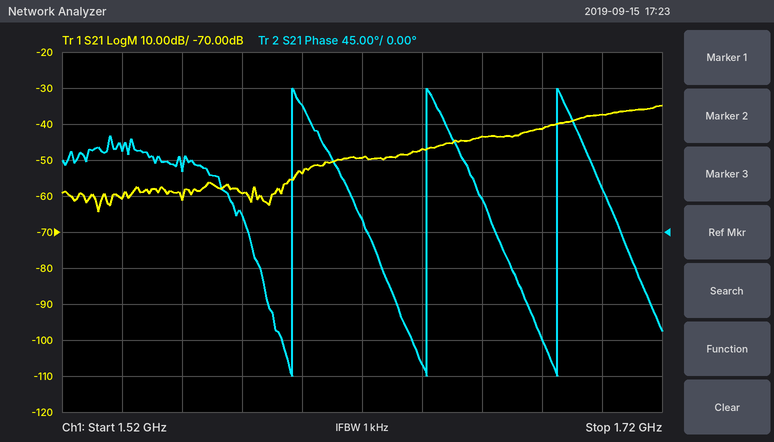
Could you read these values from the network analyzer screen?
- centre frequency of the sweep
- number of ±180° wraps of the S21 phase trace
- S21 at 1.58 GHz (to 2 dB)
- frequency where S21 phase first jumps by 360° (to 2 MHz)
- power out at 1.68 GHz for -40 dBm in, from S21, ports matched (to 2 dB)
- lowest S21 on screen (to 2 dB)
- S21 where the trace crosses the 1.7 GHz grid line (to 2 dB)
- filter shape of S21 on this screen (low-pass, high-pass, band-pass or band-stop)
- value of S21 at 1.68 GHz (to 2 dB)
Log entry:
1.62 GHz
3
-60 dB
1.596 GHz
-82 dBm
-64 dB
-38 dB
high-pass
-42 dB
